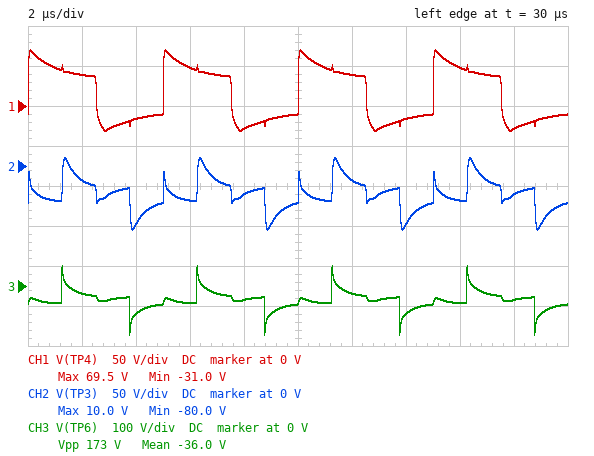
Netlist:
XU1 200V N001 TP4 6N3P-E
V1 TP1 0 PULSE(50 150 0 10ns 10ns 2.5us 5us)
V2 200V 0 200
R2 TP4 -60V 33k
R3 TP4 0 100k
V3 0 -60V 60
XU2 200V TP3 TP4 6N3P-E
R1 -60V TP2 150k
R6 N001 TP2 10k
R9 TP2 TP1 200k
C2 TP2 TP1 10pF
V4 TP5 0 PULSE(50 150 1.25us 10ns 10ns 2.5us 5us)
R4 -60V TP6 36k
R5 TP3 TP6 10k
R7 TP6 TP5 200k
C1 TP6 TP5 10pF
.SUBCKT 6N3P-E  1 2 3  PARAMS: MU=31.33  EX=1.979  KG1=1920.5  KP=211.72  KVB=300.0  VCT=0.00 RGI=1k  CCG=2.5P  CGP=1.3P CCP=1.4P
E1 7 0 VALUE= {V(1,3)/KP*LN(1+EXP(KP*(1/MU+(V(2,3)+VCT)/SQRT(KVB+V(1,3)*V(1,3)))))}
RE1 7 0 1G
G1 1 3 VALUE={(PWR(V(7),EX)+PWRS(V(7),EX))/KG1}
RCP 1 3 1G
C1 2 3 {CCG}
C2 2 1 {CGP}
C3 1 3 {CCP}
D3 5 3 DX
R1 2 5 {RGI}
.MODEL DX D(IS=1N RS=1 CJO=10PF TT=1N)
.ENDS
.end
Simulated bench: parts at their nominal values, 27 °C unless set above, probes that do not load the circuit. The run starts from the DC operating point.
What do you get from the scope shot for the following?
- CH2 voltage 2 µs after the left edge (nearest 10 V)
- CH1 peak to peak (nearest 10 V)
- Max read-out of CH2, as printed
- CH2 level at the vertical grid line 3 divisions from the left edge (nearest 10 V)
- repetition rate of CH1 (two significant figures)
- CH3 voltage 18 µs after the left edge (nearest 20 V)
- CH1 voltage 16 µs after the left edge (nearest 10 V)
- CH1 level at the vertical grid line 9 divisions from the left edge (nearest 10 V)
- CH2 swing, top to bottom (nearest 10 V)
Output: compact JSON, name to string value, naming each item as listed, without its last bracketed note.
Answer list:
{"CH2 voltage 2 µs after the left edge": "-20 V", "CH1 peak to peak": "100 V", "Max read-out of CH2, as printed": "10.0 V", "CH2 level at the vertical grid line 3 divisions from the left edge": "-40 V", "repetition rate of CH1": "200 kHz", "CH3 voltage 18 µs after the left edge": "-40 V", "CH1 voltage 16 µs after the left edge": "50 V", "CH1 level at the vertical grid line 9 divisions from the left edge": "-30 V", "CH2 swing, top to bottom": "90 V"}
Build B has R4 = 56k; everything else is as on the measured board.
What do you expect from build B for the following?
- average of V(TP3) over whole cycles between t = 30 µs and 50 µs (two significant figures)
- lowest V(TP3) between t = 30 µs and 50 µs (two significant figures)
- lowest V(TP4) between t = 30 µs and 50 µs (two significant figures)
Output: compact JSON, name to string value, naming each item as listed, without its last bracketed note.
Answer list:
{"average of V(TP3) over whole cycles between t = 30 µs and 50 µs": "-25 V", "lowest V(TP3) between t = 30 µs and 50 µs": "-72 V", "lowest V(TP4) between t = 30 µs and 50 µs": "-33 V"}
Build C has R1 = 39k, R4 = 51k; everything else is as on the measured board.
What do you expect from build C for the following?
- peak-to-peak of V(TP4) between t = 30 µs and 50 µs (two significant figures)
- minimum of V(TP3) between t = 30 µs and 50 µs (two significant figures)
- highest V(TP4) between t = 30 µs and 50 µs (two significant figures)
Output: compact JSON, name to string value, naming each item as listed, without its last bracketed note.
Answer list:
{"peak-to-peak of V(TP4) between t = 30 µs and 50 µs": "81 V", "minimum of V(TP3) between t = 30 µs and 50 µs": "-80 V", "highest V(TP4) between t = 30 µs and 50 µs": "38 V"}
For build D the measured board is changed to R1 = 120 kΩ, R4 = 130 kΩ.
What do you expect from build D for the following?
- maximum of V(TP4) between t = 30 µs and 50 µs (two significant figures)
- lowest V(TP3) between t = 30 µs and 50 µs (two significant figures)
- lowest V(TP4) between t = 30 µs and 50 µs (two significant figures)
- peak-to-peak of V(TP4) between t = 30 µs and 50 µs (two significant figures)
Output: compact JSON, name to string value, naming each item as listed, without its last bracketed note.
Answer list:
{"maximum of V(TP4) between t = 30 µs and 50 µs": "60 V", "lowest V(TP3) between t = 30 µs and 50 µs": "-50 V", "lowest V(TP4) between t = 30 µs and 50 µs": "-32 V", "peak-to-peak of V(TP4) between t = 30 µs and 50 µs": "92 V"}
